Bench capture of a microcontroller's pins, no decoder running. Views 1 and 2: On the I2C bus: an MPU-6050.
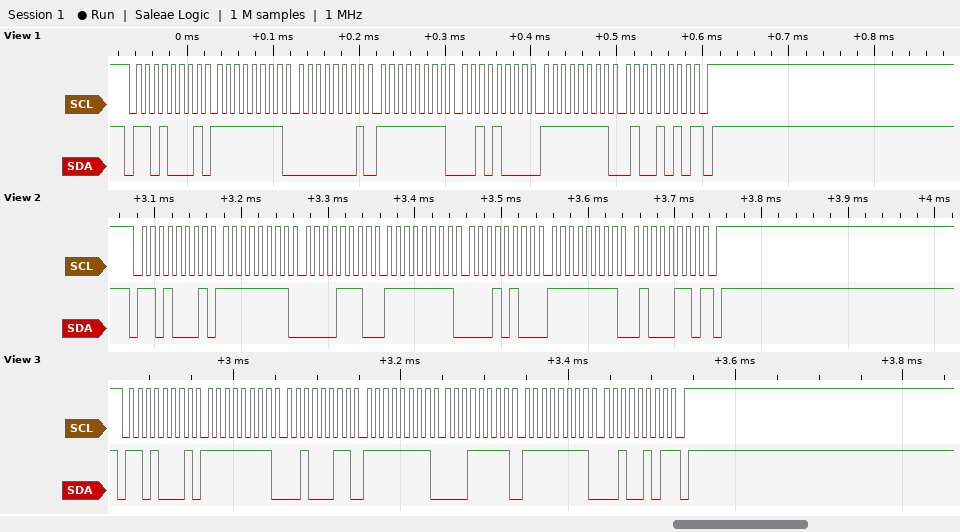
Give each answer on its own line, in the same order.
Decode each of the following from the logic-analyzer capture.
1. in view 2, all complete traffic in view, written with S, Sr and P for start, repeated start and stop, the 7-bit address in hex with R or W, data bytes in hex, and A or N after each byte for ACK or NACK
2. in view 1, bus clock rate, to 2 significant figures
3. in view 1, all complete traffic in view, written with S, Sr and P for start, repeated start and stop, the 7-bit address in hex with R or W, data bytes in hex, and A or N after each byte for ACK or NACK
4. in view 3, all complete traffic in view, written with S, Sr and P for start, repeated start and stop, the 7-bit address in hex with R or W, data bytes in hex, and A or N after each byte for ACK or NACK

S 68R A FF A 0E A FF A 14 A FF A 46 N P
100 kHz
S 68R A FF A 01 A FF A 28 A FF A 4A N P
S 68R A FF A 23 A FF A 1F A FF A 25 N P
